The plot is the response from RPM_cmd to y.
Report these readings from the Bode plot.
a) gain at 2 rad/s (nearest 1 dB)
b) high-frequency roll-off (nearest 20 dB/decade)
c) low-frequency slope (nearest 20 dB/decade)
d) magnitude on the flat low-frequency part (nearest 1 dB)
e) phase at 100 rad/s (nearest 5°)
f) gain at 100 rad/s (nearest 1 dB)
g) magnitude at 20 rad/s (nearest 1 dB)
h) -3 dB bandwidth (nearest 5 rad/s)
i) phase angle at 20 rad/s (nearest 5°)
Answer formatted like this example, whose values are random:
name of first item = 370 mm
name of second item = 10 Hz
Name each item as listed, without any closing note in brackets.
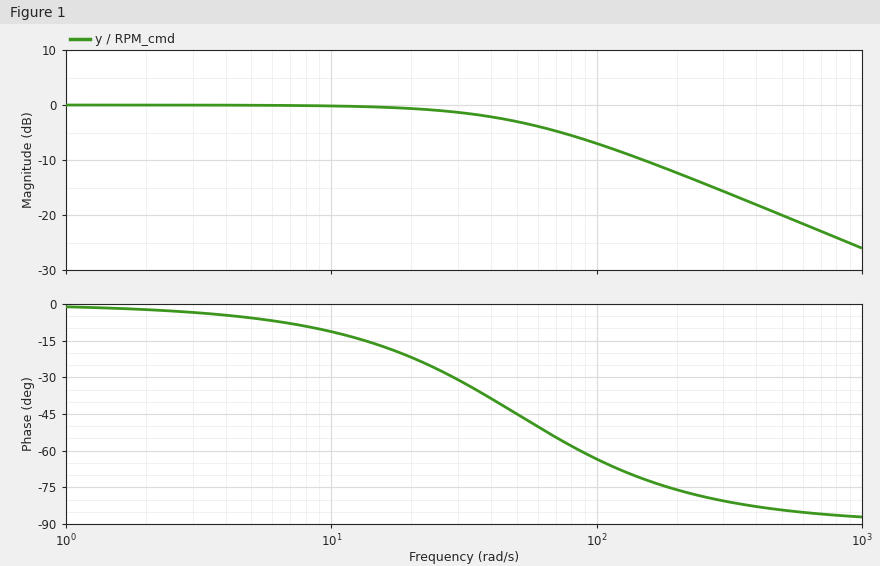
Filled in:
gain at 2 rad/s = 0 dB
high-frequency roll-off = -20 dB/decade
low-frequency slope = 0 dB/decade
magnitude on the flat low-frequency part = 0 dB
phase at 100 rad/s = -65°
gain at 100 rad/s = -7 dB
magnitude at 20 rad/s = -1 dB
-3 dB bandwidth = 50 rad/s
phase angle at 20 rad/s = -20°
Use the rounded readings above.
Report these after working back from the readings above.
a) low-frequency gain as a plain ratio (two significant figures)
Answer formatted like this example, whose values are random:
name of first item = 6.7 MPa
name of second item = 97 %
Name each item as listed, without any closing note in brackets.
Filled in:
low-frequency gain as a plain ratio = 1.0
